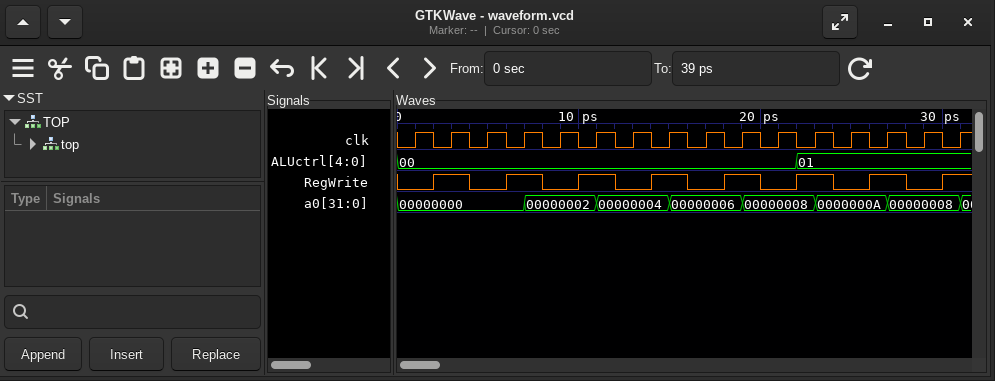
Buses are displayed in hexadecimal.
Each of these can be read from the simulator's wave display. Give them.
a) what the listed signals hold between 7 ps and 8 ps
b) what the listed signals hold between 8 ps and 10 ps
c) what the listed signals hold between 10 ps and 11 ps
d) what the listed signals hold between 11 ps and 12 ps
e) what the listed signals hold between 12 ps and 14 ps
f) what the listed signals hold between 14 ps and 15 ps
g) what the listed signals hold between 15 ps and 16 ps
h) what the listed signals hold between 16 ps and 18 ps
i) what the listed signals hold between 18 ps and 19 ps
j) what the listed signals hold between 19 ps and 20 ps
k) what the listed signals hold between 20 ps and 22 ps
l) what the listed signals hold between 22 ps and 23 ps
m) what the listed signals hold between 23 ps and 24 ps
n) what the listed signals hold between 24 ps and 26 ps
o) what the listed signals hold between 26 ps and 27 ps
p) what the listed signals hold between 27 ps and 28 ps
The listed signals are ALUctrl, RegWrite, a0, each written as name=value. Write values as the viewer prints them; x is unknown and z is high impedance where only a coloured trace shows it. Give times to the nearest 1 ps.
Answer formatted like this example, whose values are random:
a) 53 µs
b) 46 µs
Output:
a) ALUctrl=00, RegWrite=1, a0=00000002
b) ALUctrl=00, RegWrite=0, a0=00000002
c) ALUctrl=00, RegWrite=1, a0=00000002
d) ALUctrl=00, RegWrite=1, a0=00000004
e) ALUctrl=00, RegWrite=0, a0=00000004
f) ALUctrl=00, RegWrite=1, a0=00000004
g) ALUctrl=00, RegWrite=1, a0=00000006
h) ALUctrl=00, RegWrite=0, a0=00000006
i) ALUctrl=00, RegWrite=1, a0=00000006
j) ALUctrl=00, RegWrite=1, a0=00000008
k) ALUctrl=00, RegWrite=0, a0=00000008
l) ALUctrl=01, RegWrite=1, a0=00000008
m) ALUctrl=01, RegWrite=1, a0=0000000A
n) ALUctrl=01, RegWrite=0, a0=0000000A
o) ALUctrl=01, RegWrite=1, a0=0000000A
p) ALUctrl=01, RegWrite=1, a0=00000008
